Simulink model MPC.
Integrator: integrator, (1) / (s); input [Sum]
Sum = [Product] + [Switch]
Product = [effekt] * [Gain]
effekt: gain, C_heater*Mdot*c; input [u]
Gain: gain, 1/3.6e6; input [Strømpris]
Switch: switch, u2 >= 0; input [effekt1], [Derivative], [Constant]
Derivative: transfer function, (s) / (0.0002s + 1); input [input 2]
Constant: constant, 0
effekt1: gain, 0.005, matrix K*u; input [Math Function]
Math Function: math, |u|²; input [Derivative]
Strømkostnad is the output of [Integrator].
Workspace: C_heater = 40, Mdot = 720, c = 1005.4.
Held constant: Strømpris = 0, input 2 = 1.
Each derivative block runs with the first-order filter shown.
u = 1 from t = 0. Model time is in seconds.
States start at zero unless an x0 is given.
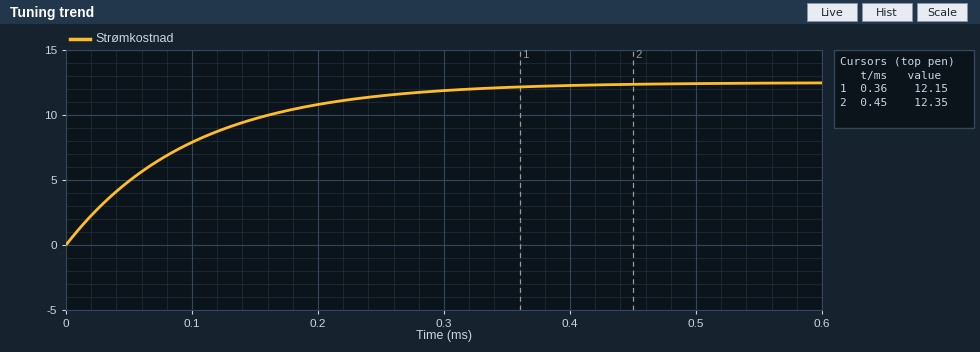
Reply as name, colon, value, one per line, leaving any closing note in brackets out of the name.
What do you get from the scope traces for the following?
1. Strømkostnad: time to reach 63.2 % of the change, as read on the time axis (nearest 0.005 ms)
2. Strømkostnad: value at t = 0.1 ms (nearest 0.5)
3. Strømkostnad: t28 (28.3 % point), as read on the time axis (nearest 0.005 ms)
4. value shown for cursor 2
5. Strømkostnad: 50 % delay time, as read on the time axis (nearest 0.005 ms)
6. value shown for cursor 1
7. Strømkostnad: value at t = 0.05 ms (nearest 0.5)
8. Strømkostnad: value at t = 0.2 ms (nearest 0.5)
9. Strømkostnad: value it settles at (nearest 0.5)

Strømkostnad: time to reach 63.2 % of the change, as read on the time axis: 0.100 ms
Strømkostnad: value at t = 0.1 ms: 8.0
Strømkostnad: t28 (28.3 % point), as read on the time axis: 0.035 ms
value shown for cursor 2: 12.35
Strømkostnad: 50 % delay time, as read on the time axis: 0.070 ms
value shown for cursor 1: 12.15
Strømkostnad: value at t = 0.05 ms: 5.0
Strømkostnad: value at t = 0.2 ms: 11.0
Strømkostnad: value it settles at: 12.5
